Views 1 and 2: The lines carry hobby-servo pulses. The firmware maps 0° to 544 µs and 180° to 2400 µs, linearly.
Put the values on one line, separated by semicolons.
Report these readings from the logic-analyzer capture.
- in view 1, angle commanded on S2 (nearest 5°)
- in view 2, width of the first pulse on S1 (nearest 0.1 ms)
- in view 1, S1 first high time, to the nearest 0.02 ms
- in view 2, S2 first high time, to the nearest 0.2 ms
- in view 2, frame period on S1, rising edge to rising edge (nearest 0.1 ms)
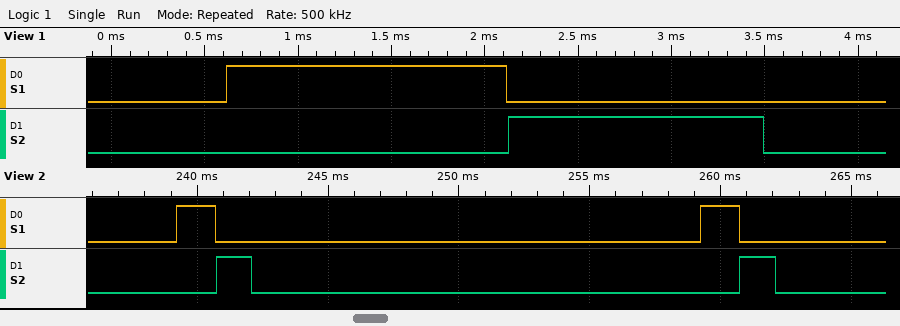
80°; 1.5 ms; 1.50 ms; 1.4 ms; 20.0 ms
